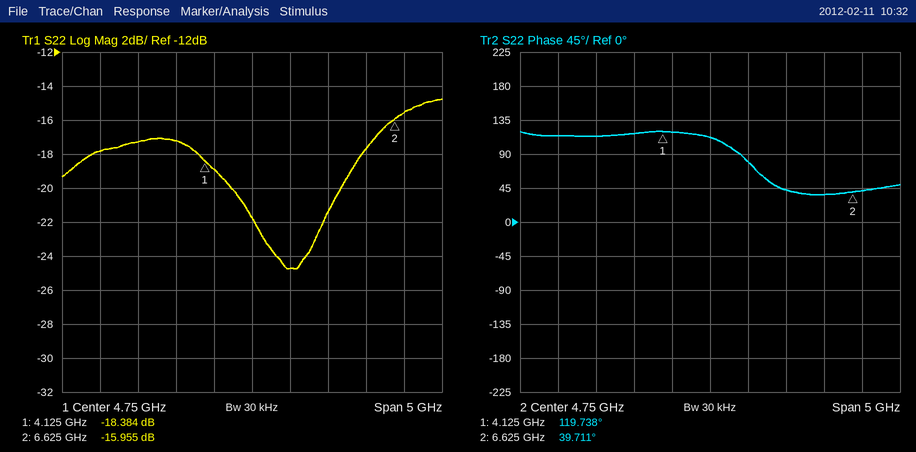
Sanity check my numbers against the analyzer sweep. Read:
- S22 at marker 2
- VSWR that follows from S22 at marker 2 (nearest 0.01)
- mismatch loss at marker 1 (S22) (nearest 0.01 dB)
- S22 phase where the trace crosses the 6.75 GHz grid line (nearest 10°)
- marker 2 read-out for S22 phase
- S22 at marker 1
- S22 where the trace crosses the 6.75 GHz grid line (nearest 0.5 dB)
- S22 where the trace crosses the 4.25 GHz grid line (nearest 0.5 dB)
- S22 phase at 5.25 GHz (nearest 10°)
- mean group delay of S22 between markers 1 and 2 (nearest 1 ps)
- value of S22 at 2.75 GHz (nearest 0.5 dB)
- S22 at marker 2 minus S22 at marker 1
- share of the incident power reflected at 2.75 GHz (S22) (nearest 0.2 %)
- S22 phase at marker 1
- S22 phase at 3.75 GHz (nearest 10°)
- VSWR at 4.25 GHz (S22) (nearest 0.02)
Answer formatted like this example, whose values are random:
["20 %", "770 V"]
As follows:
["-15.955 dB", "1.38", "0.06 dB", "40°", "39.711°", "-18.384 dB", "-15.5 dB", "-19.0 dB", "80°", "89 ps", "-18.0 dB", "2.429 dB", "1.6 %", "119.738°", "120°", "1.26"]
